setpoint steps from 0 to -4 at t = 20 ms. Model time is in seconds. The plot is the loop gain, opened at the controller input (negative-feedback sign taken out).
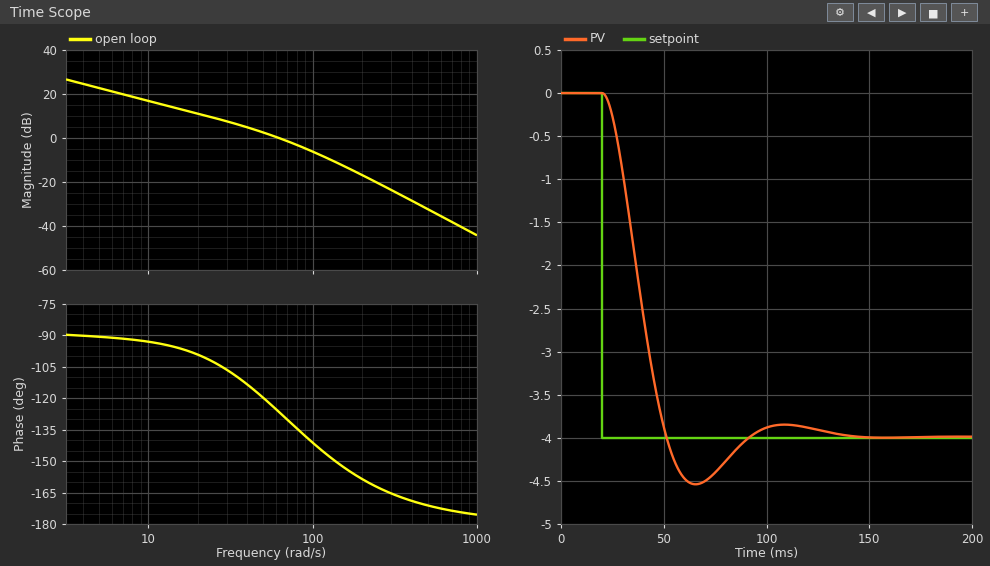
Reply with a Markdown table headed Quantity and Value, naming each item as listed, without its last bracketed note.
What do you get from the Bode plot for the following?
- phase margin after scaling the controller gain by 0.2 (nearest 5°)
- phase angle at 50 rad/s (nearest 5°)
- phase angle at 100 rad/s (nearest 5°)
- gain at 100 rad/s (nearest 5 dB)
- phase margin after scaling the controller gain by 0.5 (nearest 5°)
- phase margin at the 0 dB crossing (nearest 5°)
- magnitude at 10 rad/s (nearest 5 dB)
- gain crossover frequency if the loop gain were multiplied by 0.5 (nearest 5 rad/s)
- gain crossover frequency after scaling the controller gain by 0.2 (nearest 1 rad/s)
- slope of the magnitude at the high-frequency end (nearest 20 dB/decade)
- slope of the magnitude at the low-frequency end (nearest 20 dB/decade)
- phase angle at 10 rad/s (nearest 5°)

| Quantity | Value |
|---|---|
| phase margin after scaling the controller gain by 0.2 | 85° |
| phase angle at 50 rad/s | -120° |
| phase angle at 100 rad/s | -140° |
| gain at 100 rad/s | -5 dB |
| phase margin after scaling the controller gain by 0.5 | 70° |
| phase margin at the 0 dB crossing | 55° |
| magnitude at 10 rad/s | 15 dB |
| gain crossover frequency if the loop gain were multiplied by 0.5 | 35 rad/s |
| gain crossover frequency after scaling the controller gain by 0.2 | 14 rad/s |
| slope of the magnitude at the high-frequency end | -40 dB/decade |
| slope of the magnitude at the low-frequency end | -20 dB/decade |
| phase angle at 10 rad/s | -95° |
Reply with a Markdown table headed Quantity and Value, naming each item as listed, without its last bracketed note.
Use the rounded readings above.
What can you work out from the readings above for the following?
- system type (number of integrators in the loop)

| Quantity | Value |
|---|---|
| system type | 1 |
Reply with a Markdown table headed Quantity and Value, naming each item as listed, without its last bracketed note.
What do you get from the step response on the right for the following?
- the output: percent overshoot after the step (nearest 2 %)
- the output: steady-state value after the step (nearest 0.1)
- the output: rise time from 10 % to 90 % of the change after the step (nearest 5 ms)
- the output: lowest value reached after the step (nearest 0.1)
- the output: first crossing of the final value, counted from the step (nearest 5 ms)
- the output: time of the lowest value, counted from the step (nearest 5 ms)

| Quantity | Value |
|---|---|
| the output: percent overshoot after the step | 14 % |
| the output: steady-state value after the step | -4.0 |
| the output: rise time from 10 % to 90 % of the change after the step | 20 ms |
| the output: lowest value reached after the step | -4.5 |
| the output: first crossing of the final value, counted from the step | 30 ms |
| the output: time of the lowest value, counted from the step | 45 ms |
